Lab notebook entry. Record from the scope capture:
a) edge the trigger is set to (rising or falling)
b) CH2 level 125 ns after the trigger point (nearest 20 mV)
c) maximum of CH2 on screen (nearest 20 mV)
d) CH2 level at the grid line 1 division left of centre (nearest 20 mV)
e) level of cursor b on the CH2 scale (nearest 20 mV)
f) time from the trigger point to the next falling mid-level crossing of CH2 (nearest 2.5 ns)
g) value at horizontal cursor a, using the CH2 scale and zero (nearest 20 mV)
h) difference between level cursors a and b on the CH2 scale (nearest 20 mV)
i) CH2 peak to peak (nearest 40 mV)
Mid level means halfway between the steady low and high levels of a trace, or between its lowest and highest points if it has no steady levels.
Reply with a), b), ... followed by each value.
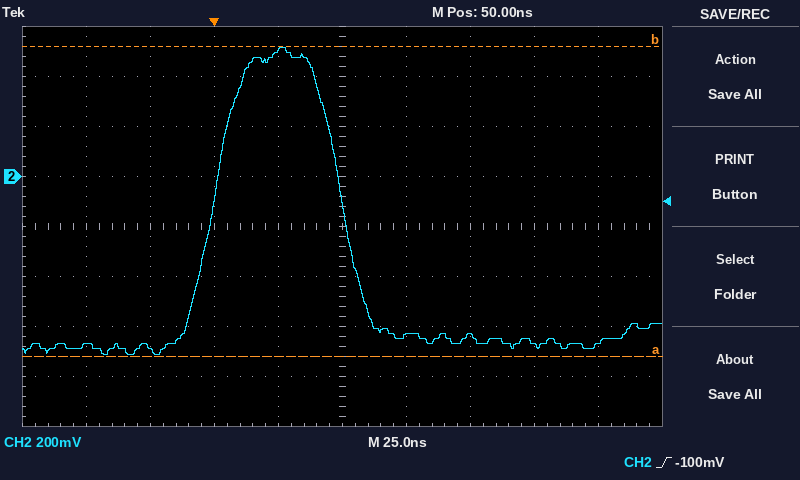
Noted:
a) rising
b) -680 mV
c) 520 mV
d) 500 mV
e) 520 mV
f) 50.0 ns
g) -720 mV
h) 1.24 V
i) 1.24 V
